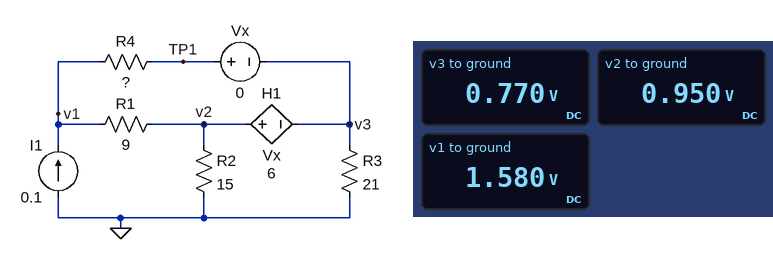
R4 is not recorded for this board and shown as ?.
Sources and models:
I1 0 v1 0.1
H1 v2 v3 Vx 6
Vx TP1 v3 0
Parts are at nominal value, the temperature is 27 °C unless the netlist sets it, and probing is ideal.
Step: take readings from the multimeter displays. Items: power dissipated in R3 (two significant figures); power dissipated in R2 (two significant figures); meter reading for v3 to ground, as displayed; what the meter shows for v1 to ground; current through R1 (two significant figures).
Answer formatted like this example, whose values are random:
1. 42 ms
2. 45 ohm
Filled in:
1. 28 mW
2. 60 mW
3. 0.770 V
4. 1.580 V
5. 70 mA
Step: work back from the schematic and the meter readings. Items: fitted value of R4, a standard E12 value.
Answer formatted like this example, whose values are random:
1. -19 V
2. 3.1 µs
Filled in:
1. 27 Ω
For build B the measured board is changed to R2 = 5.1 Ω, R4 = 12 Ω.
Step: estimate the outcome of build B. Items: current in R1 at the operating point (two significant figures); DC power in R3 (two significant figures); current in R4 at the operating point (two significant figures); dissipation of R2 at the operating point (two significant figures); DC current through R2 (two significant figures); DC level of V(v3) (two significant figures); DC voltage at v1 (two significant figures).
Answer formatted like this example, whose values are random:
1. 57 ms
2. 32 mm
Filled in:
1. 40 mA
2. 690 µW
3. 60 mA
4. 45 mW
5. 94 mA
6. 120 mV
7. 840 mV
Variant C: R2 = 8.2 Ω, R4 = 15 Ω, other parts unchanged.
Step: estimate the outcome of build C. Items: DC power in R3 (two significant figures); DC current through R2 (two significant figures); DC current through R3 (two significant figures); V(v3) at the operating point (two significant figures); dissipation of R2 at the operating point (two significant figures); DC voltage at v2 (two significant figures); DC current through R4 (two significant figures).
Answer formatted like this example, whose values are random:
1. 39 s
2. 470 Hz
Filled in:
1. 6.7 mW
2. 82 mA
3. 18 mA
4. 370 mV
5. 55 mW
6. 670 mV
7. 50 mA
